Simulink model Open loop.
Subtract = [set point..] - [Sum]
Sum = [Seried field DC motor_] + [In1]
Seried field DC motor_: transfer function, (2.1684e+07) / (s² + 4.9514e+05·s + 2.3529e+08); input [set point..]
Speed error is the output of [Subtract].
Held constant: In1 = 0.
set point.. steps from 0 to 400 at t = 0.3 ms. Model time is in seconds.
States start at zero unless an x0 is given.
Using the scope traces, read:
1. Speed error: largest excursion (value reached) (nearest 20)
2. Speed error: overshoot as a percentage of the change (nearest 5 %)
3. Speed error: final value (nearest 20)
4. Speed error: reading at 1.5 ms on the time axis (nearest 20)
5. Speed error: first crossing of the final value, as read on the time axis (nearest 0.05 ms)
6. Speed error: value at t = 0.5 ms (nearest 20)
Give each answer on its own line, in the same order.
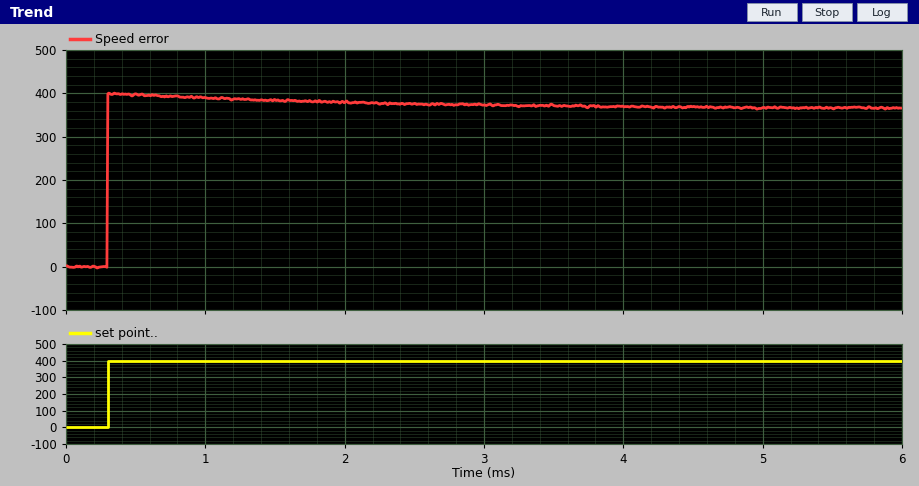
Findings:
400
10 %
360
380
0.30 ms
400
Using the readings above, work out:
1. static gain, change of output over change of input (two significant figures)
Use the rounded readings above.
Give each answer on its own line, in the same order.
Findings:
0.90
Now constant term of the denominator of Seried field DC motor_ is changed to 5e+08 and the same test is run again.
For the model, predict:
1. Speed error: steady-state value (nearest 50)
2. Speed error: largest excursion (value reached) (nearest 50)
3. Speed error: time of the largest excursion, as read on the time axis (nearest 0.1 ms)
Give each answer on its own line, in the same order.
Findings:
400
400
0.3 ms
